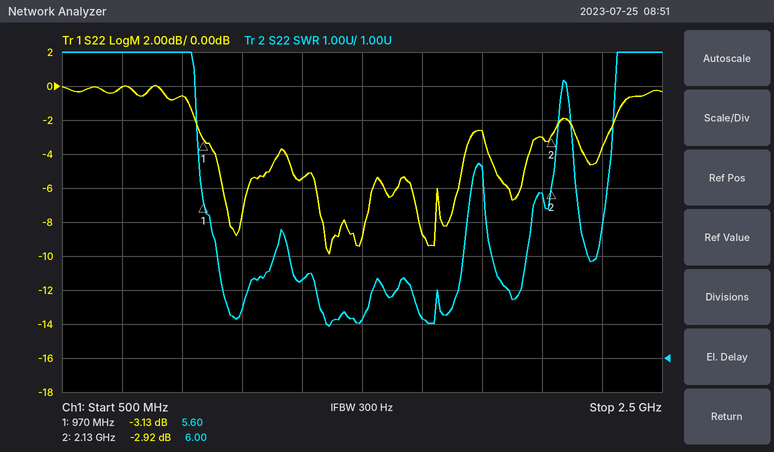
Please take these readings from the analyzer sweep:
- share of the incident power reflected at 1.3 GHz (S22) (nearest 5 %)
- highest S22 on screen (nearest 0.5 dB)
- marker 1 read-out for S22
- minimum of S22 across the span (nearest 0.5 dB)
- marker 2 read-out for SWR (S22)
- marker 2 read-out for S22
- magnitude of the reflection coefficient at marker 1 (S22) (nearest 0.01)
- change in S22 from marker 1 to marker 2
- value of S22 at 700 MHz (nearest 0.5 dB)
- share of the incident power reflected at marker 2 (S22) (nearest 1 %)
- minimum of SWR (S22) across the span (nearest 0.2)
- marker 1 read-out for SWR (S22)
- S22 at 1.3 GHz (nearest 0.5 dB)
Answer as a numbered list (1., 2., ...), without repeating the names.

1. 30 %
2. 0.0 dB
3. -3.13 dB
4. -10.0 dB
5. 6.00
6. -2.92 dB
7. 0.70
8. 0.21 dB
9. 0.0 dB
10. 51 %
11. 2.0
12. 5.60
13. -5.5 dB
